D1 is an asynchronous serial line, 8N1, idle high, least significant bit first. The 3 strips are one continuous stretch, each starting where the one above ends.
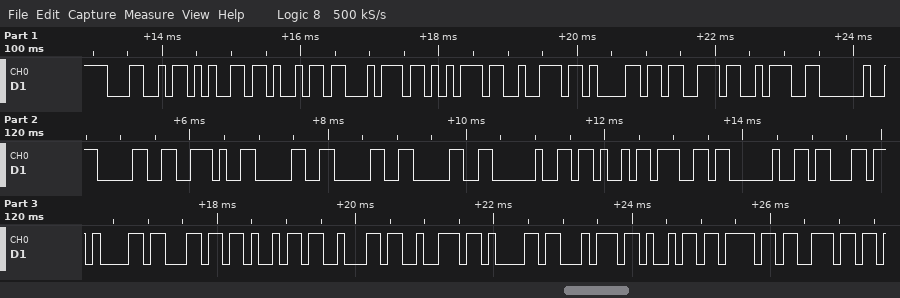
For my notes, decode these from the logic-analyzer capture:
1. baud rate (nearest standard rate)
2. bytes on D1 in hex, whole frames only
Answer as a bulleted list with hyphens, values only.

- 9600 baud
- 0x4C 0x65 0x69 0x74 0x75 0x72 0x61 0x73 0x3A 0x20 0x30 0x2E 0x30 0x30 0x30 0x20 0x4B 0x67 0x20 0x63 0x61 0x6C 0x69 0x62 0x72 0x61 0x74 0x69 0x6F 0x6E
